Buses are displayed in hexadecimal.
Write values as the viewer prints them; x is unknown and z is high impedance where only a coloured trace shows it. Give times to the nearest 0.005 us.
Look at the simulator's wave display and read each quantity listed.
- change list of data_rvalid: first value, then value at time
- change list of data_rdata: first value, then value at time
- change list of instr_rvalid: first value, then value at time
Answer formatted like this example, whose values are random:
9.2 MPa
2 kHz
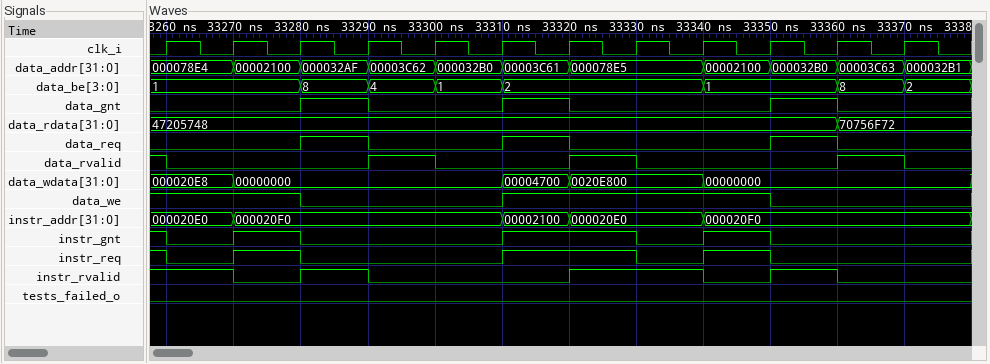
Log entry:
1, 0 at 33.26 us, 1 at 33.29 us, 0 at 33.3 us, 1 at 33.32 us, 0 at 33.33 us, 1 at 33.36 us, 0 at 33.37 us
47205748, 70756F72 at 33.36 us
1, 0 at 33.27 us, 1 at 33.28 us, 0 at 33.29 us, 1 at 33.32 us, 0 at 33.34 us, 1 at 33.35 us, 0 at 33.36 us
